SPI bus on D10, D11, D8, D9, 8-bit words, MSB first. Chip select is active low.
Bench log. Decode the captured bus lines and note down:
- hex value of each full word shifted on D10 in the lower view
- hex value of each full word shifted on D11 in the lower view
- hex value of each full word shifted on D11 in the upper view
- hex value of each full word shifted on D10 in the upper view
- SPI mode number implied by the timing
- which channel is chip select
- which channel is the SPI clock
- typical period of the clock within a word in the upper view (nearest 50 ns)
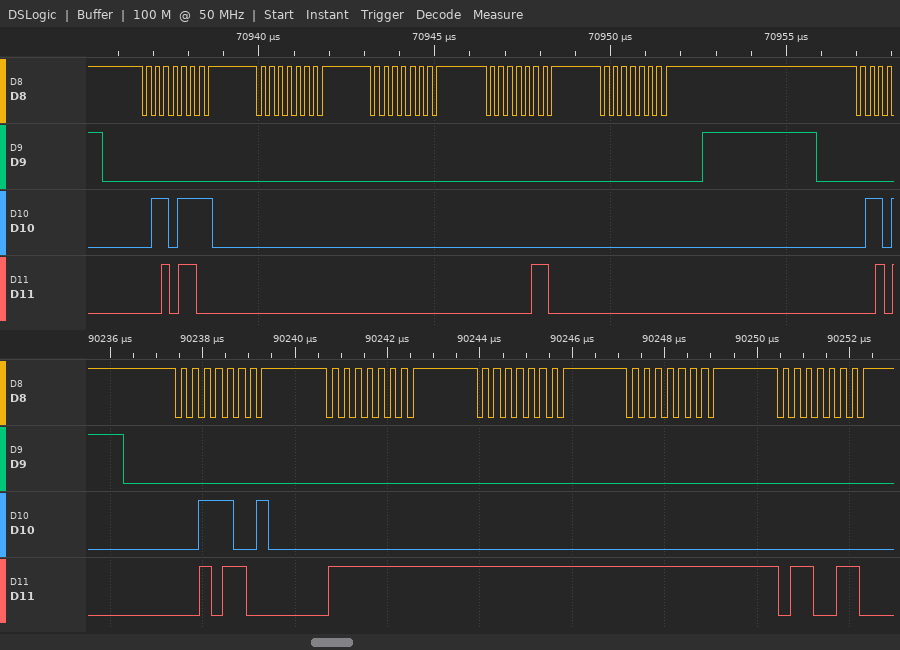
39, 00, 00, 00, 00
2C, FF, FF, FF, 66
2C, 00, 00, 06, 00
6F, 00, 00, 00, 00
3
D9
D8
250 ns
